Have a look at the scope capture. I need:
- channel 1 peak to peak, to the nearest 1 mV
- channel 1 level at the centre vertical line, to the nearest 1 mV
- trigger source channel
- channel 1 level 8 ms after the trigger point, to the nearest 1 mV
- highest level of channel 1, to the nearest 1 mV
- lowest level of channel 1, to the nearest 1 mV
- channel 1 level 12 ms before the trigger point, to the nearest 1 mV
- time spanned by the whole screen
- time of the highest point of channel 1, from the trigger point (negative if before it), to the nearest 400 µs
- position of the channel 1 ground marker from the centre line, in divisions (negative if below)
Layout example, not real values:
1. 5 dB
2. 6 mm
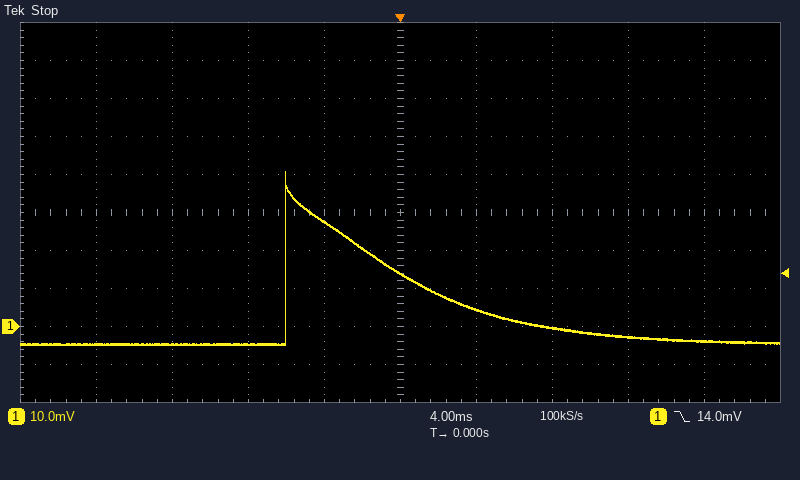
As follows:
1. 46 mV
2. 14 mV
3. channel 1
4. 0 mV
5. 41 mV
6. -5 mV
7. -5 mV
8. 40 ms
9. -6.0 ms
10. -3.0 div
